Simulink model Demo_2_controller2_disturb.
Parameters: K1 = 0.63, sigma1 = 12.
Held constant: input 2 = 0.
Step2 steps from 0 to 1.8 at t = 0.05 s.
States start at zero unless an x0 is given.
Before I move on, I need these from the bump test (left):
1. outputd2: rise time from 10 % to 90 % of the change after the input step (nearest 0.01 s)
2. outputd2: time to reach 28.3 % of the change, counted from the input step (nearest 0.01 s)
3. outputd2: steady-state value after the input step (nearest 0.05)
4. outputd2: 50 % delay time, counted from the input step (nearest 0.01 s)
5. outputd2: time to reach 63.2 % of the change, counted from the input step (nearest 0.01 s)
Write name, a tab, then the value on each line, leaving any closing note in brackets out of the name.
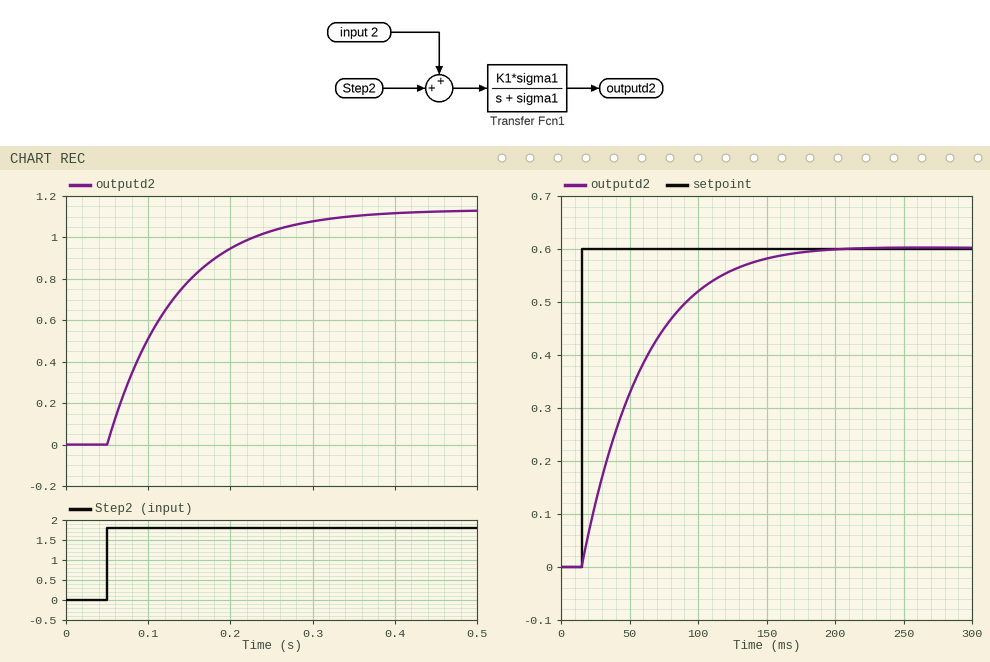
outputd2: rise time from 10 % to 90 % of the change after the input step	0.18 s
outputd2: time to reach 28.3 % of the change, counted from the input step	0.03 s
outputd2: steady-state value after the input step	1.15
outputd2: 50 % delay time, counted from the input step	0.06 s
outputd2: time to reach 63.2 % of the change, counted from the input step	0.08 s
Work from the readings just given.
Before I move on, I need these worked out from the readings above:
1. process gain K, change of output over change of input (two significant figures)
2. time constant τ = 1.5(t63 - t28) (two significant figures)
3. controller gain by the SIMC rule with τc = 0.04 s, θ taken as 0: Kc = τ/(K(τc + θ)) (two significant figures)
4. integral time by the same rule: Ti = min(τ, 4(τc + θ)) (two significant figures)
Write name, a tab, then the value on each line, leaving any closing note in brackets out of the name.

process gain K, change of output over change of input	0.64
time constant τ = 1.5(t63 - t28)	0.075 s
controller gain by the SIMC rule with τc = 0.04 s, θ taken as 0: Kc = τ/(K(τc + θ))	2.9
integral time by the same rule: Ti = min(τ, 4(τc + θ))	0.075 s
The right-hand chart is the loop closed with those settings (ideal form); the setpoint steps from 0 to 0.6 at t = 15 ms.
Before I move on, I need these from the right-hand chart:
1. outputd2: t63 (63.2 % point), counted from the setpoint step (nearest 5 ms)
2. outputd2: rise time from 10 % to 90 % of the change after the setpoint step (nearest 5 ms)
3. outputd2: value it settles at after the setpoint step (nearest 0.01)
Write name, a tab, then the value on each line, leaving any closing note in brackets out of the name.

outputd2: t63 (63.2 % point), counted from the setpoint step	45 ms
outputd2: rise time from 10 % to 90 % of the change after the setpoint step	90 ms
outputd2: value it settles at after the setpoint step	0.60
